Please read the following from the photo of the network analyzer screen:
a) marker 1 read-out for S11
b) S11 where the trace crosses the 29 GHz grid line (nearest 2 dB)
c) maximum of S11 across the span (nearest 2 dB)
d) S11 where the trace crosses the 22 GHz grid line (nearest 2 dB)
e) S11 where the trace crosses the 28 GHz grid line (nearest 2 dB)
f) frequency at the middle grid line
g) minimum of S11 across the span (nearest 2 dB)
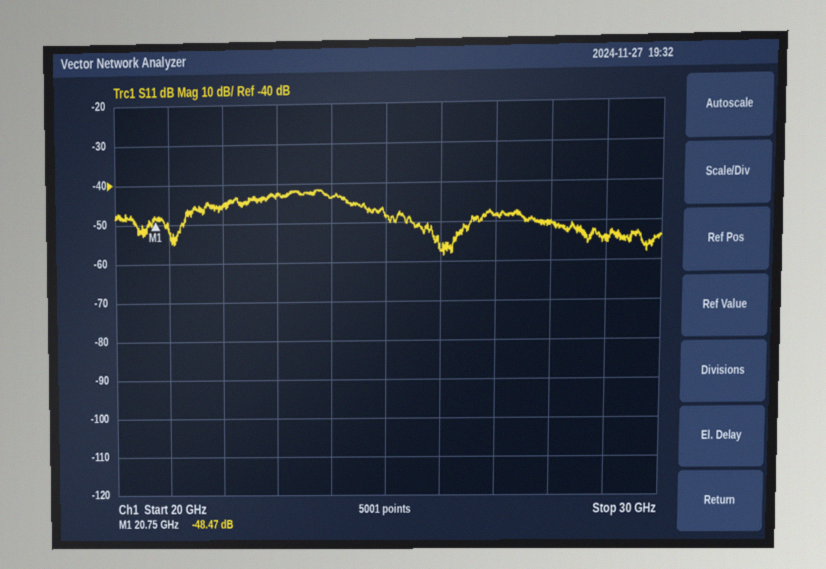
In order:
-48.47 dB
-54 dB
-42 dB
-46 dB
-50 dB
25 GHz
-58 dB
